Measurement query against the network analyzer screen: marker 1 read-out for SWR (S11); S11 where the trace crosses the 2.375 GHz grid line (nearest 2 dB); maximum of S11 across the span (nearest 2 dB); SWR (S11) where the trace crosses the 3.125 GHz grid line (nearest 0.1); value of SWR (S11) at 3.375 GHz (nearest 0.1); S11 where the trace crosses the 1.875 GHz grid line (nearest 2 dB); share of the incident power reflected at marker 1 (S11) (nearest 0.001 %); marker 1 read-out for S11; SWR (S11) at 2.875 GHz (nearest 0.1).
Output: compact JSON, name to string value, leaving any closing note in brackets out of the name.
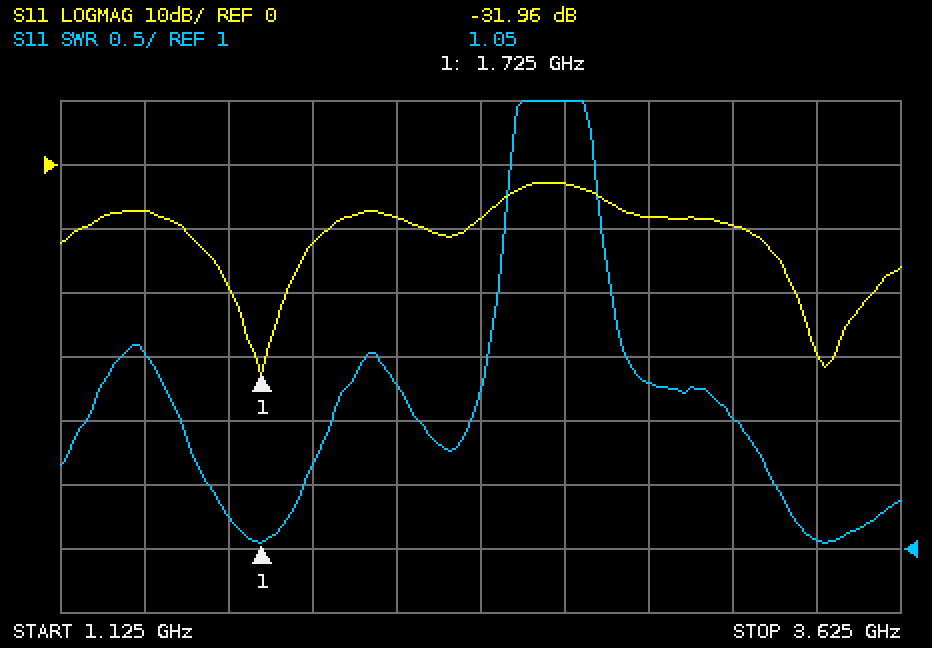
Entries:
{"marker 1 read-out for SWR": "1.05", "S11 where the trace crosses the 2.375 GHz grid line": "-8 dB", "maximum of S11 across the span": "-2 dB", "SWR (S11) where the trace crosses the 3.125 GHz grid line": "2.0", "value of SWR (S11) at 3.375 GHz": "1.1", "S11 where the trace crosses the 1.875 GHz grid line": "-12 dB", "share of the incident power reflected at marker 1 (S11)": "0.064 %", "marker 1 read-out for S11": "-31.96 dB", "SWR (S11) at 2.875 GHz": "2.3"}
